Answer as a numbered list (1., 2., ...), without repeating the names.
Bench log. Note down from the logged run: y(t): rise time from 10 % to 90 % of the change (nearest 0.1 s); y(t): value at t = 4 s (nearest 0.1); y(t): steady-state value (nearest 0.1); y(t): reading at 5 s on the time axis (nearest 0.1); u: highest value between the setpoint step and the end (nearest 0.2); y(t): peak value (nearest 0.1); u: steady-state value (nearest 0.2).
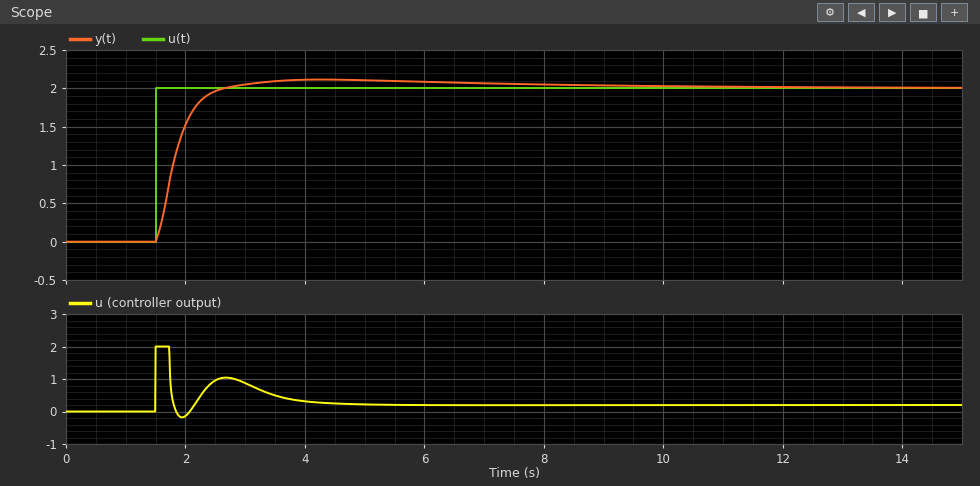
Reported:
1. 0.6 s
2. 2.1
3. 2.0
4. 2.1
5. 2.0
6. 2.1
7. 0.2
